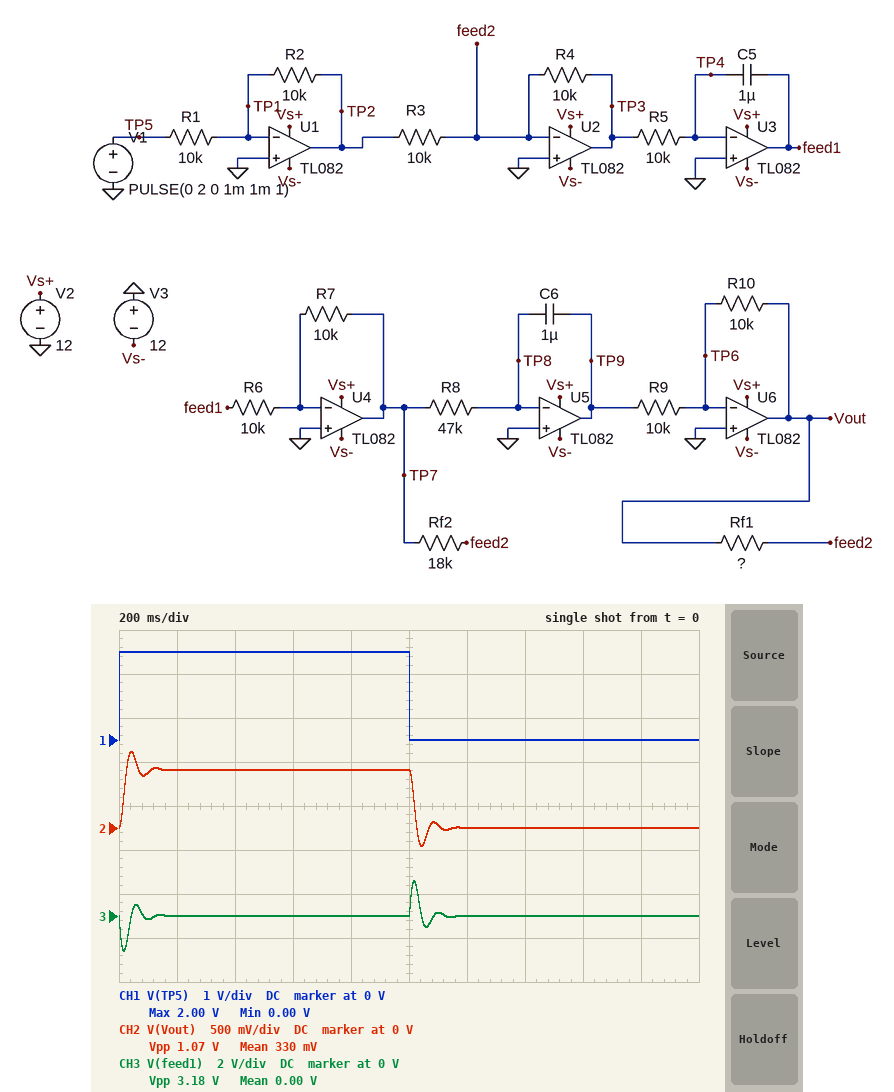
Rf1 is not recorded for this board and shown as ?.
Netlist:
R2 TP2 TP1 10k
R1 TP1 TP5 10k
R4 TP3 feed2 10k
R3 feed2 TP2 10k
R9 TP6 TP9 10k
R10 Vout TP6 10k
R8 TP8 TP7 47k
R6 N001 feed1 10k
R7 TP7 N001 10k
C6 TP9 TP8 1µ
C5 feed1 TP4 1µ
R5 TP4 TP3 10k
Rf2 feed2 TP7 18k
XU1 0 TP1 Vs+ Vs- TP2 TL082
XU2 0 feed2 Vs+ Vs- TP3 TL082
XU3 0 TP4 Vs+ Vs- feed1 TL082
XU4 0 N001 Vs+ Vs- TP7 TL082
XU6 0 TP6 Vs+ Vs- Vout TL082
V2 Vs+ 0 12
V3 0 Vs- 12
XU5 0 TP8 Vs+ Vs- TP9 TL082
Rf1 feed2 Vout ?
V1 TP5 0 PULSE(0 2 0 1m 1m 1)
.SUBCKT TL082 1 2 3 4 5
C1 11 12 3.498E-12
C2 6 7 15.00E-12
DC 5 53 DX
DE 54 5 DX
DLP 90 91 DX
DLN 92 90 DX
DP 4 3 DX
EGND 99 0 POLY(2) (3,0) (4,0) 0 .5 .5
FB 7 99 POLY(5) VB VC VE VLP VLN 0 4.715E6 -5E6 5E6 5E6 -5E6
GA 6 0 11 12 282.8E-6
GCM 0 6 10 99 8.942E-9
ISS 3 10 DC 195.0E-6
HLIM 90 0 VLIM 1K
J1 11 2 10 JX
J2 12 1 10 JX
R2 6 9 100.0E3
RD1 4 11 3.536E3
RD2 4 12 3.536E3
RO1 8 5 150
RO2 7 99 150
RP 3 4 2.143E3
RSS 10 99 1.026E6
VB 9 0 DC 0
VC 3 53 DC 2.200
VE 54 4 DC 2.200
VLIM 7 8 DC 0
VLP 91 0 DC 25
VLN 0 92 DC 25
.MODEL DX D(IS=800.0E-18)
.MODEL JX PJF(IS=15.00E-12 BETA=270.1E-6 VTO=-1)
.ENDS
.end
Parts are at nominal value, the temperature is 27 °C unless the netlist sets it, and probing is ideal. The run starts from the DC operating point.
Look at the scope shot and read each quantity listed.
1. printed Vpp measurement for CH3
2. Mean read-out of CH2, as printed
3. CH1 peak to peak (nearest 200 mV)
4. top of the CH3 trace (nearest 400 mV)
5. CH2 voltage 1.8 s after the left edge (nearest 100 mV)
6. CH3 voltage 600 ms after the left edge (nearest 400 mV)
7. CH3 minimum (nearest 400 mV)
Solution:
3.18 V
330 mV
2.0 V
1.6 V
0 V
0 V
-1.6 V
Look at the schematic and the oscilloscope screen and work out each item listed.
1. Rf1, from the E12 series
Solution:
3.3 kΩ
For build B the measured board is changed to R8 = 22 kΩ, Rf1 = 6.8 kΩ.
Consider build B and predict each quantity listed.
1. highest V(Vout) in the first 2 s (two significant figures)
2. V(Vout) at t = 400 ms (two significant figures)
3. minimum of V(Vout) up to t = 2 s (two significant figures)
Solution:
1.8 V
1.4 V
-440 mV
